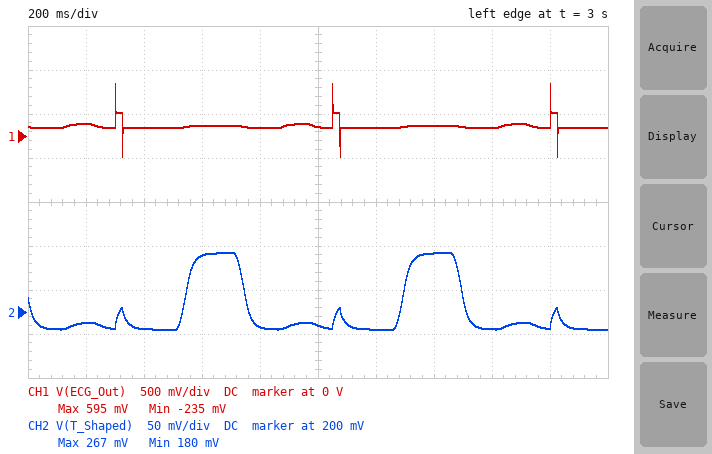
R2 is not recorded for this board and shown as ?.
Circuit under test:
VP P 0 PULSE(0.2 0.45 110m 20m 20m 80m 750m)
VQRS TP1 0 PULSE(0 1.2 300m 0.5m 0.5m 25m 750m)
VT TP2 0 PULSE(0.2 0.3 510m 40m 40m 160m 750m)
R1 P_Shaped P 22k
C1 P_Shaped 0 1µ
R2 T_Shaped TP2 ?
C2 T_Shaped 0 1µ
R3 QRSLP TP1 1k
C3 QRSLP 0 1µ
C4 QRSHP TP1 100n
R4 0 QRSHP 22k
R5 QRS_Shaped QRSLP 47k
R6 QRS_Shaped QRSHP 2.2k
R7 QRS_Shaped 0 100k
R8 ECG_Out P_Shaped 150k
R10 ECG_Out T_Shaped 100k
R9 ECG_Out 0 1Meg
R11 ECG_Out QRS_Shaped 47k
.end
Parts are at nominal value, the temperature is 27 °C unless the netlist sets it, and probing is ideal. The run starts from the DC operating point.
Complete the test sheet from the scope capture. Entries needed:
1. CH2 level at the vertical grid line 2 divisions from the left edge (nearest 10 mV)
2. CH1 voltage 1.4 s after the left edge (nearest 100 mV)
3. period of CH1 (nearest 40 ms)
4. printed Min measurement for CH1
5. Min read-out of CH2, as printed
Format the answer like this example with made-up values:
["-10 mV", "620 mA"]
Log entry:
["180 mV", "100 mV", "760 ms", "-235 mV", "180 mV"]
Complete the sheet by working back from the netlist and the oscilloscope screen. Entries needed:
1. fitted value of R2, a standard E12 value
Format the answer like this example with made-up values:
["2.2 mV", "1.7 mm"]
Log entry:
["22 kΩ"]
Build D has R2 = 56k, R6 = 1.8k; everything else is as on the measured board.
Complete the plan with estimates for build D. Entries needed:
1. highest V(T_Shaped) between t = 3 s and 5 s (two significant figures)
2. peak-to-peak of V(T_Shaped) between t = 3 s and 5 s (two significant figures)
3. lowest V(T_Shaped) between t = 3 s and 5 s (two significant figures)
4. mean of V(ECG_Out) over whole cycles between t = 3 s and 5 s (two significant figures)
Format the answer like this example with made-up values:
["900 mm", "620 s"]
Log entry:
["230 mV", "71 mV", "160 mV", "100 mV"]
